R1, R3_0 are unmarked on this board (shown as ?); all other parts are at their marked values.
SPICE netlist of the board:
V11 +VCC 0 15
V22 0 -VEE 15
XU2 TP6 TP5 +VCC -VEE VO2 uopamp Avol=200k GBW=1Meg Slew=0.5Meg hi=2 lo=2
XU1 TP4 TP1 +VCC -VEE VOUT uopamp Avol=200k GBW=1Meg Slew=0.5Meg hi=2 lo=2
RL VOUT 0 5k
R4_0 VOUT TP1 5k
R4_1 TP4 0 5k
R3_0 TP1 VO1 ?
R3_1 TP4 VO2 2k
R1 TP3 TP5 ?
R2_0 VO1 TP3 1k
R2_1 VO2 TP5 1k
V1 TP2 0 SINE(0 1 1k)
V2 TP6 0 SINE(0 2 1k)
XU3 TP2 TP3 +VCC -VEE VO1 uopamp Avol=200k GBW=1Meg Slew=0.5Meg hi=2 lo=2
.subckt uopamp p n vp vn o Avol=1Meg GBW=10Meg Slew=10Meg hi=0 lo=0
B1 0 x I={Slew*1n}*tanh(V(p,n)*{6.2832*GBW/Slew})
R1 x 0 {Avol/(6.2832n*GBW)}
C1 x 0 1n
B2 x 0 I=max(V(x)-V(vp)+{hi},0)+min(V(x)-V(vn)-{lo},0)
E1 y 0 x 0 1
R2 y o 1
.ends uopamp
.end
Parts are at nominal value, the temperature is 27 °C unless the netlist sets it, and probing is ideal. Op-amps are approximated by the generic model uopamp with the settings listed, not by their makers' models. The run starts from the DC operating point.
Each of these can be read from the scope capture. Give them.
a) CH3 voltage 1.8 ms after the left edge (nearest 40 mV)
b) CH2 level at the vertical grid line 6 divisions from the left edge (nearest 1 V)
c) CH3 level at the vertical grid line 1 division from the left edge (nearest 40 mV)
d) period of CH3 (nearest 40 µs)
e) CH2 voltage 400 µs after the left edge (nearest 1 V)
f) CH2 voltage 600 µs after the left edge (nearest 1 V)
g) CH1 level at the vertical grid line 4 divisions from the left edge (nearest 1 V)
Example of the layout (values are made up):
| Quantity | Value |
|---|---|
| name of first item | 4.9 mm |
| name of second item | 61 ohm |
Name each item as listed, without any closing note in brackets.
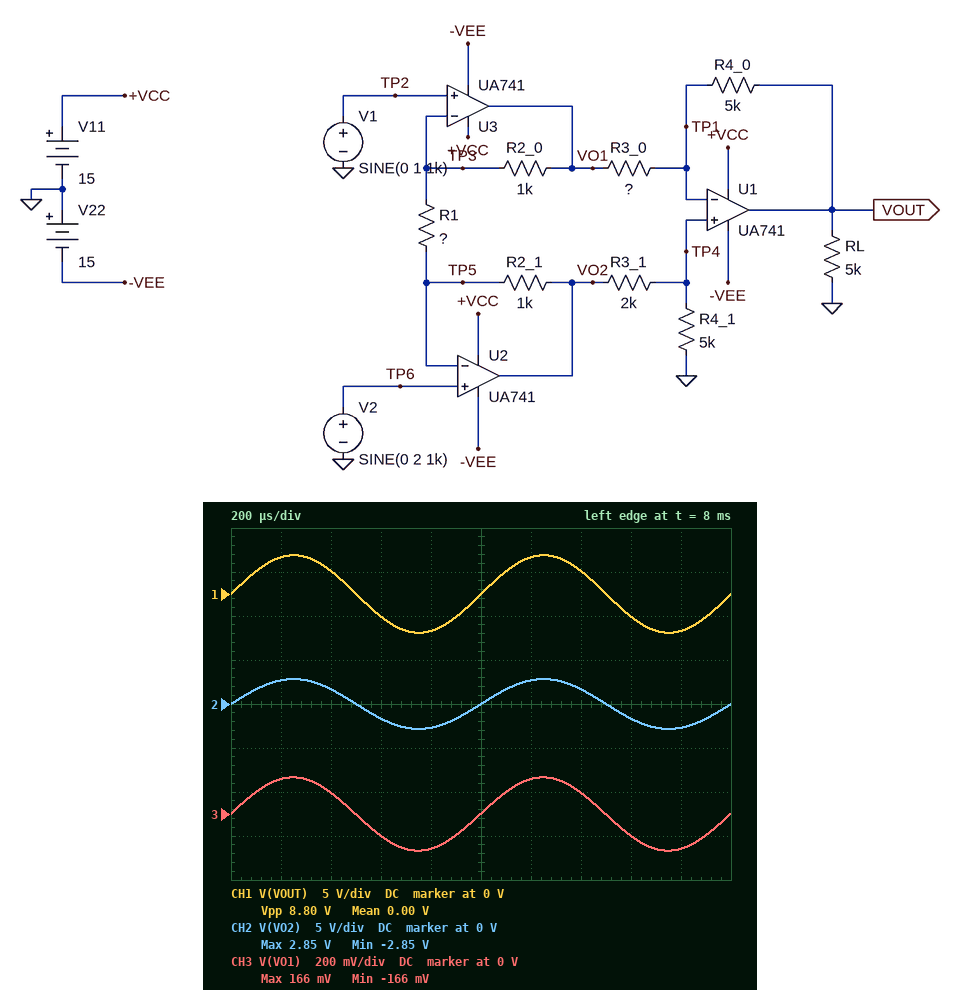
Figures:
| Quantity | Value |
|---|---|
| CH3 voltage 1.8 ms after the left edge | -160 mV |
| CH2 level at the vertical grid line 6 divisions from the left edge | 3 V |
| CH3 level at the vertical grid line 1 division from the left edge | 160 mV |
| period of CH3 | 1.00 ms |
| CH2 voltage 400 µs after the left edge | 2 V |
| CH2 voltage 600 µs after the left edge | -2 V |
| CH1 level at the vertical grid line 4 divisions from the left edge | -4 V |
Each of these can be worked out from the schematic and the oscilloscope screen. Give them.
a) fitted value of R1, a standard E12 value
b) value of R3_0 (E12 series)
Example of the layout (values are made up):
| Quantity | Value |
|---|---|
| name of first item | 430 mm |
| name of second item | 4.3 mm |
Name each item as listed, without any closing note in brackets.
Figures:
| Quantity | Value |
|---|---|
| fitted value of R1, a standard E12 value | 1.2 kΩ |
| value of R3_0 | 3.9 kΩ |
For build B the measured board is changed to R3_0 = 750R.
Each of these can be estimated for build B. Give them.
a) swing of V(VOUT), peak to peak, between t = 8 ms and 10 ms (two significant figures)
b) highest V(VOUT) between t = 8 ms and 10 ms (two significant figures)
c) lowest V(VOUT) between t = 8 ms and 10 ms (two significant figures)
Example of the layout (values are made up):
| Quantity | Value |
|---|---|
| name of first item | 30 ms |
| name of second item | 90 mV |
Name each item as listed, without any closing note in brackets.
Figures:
| Quantity | Value |
|---|---|
| swing of V(VOUT), peak to peak, between t = 8 ms and 10 ms | 26 V |
| highest V(VOUT) between t = 8 ms and 10 ms | 13 V |
| lowest V(VOUT) between t = 8 ms and 10 ms | -13 V |
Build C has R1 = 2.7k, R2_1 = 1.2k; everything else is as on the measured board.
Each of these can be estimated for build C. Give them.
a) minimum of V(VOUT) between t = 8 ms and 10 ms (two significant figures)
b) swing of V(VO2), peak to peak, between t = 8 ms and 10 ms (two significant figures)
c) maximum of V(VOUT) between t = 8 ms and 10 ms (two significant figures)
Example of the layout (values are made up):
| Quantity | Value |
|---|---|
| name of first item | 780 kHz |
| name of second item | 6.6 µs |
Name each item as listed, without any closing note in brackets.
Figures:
| Quantity | Value |
|---|---|
| minimum of V(VOUT) between t = 8 ms and 10 ms | -3.2 V |
| swing of V(VO2), peak to peak, between t = 8 ms and 10 ms | 4.9 V |
| maximum of V(VOUT) between t = 8 ms and 10 ms | 3.2 V |
